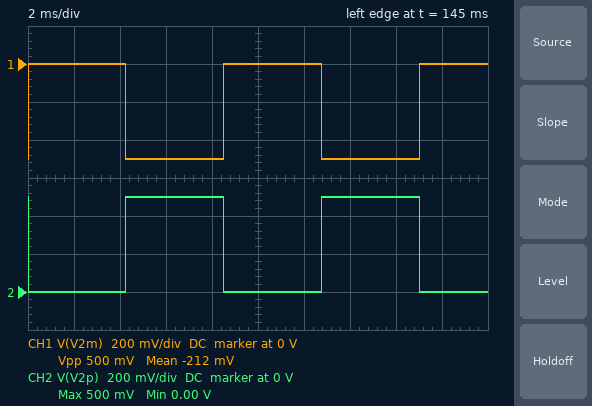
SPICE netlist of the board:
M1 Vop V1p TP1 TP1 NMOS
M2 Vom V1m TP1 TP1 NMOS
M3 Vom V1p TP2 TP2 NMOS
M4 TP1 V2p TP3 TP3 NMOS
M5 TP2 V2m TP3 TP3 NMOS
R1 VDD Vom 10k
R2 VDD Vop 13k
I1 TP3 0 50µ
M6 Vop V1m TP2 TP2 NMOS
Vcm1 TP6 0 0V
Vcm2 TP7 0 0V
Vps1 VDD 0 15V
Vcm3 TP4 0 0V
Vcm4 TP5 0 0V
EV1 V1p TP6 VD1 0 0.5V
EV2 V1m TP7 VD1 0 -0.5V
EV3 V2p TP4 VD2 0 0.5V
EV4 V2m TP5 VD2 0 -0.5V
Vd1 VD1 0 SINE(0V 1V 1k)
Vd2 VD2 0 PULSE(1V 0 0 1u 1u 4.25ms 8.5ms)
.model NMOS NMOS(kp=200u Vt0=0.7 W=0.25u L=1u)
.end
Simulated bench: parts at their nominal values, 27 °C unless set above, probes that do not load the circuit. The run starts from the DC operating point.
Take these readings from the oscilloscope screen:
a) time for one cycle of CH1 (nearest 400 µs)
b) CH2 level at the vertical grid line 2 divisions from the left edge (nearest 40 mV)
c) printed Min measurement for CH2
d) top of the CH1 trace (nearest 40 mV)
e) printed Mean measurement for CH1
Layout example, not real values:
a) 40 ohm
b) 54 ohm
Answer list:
a) 8.4 ms
b) 0 V
c) 0.00 V
d) 0 V
e) -212 mV
